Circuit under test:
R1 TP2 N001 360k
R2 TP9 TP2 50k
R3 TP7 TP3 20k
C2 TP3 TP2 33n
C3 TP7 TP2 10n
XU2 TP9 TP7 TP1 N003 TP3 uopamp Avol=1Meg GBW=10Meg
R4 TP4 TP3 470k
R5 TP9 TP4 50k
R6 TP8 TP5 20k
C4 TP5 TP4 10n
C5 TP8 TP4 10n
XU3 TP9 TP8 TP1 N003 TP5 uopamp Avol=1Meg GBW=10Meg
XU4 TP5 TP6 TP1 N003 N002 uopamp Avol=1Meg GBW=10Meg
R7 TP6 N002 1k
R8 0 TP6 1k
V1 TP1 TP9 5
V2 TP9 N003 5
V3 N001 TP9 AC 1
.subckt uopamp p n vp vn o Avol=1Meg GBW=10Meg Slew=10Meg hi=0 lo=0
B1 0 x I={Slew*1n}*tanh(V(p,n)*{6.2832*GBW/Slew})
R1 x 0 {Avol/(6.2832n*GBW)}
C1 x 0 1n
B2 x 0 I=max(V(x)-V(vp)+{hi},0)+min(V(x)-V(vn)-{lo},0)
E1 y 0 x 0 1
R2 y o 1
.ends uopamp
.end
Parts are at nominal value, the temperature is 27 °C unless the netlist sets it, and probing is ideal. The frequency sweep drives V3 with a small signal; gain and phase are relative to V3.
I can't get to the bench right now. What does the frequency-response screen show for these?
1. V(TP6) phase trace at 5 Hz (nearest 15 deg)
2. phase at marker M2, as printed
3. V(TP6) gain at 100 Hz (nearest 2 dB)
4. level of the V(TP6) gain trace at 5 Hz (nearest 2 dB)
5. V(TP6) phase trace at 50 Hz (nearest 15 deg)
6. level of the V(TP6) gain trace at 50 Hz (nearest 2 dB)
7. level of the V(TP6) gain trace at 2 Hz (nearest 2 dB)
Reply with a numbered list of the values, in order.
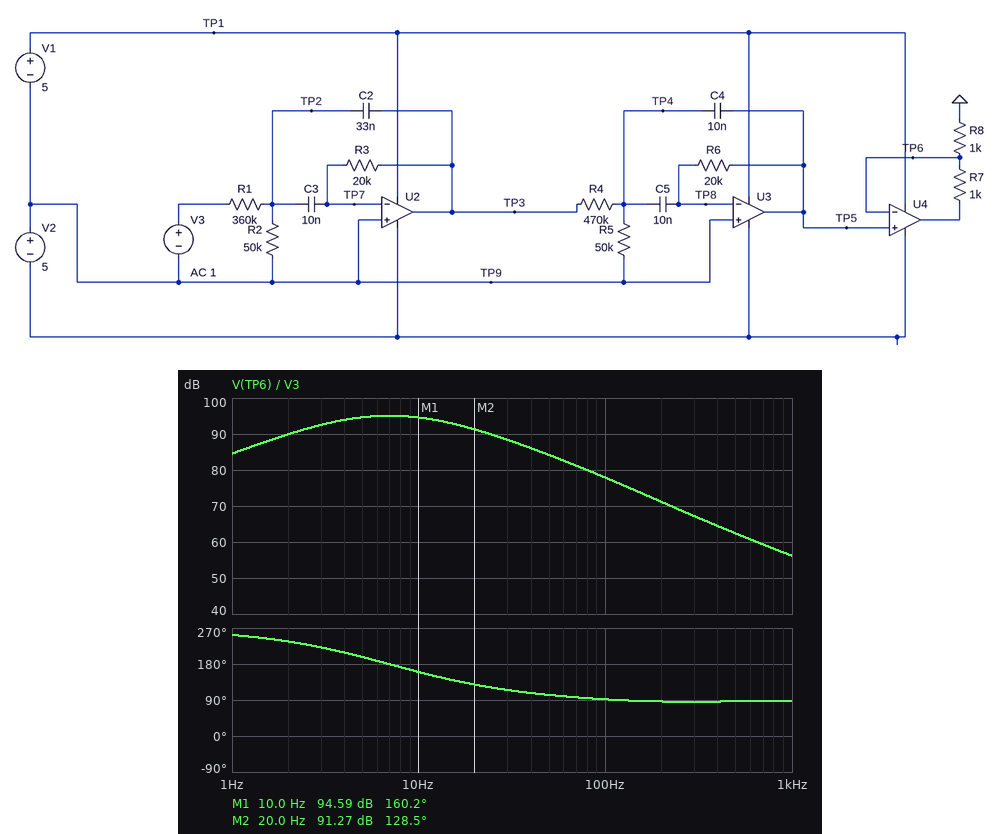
1. 195 deg
2. 128.5 deg
3. 78 dB
4. 94 dB
5. 105 deg
6. 84 dB
7. 90 dB
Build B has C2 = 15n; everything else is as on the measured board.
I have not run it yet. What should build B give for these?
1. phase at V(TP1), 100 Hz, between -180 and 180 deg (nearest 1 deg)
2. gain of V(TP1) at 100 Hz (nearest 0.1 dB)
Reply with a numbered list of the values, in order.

1. 98 deg
2. 76.8 dB
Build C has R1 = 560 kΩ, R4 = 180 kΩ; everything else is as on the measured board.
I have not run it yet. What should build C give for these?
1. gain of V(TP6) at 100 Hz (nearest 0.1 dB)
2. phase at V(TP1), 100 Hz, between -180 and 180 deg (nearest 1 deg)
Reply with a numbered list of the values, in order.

1. 74.5 dB
2. 95 deg
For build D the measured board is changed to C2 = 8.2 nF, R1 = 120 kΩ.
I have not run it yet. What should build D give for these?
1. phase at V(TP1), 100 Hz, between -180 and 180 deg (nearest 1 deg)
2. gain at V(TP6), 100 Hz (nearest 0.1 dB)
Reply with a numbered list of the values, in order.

1. 104 deg
2. 83.7 dB
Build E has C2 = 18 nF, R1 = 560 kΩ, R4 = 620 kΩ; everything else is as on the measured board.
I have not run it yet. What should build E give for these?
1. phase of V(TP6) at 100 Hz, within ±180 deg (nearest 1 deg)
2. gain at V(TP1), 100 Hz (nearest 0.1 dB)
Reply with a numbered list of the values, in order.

1. 95 deg
2. 73.5 dB
